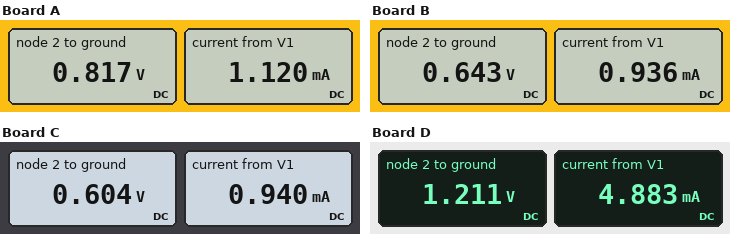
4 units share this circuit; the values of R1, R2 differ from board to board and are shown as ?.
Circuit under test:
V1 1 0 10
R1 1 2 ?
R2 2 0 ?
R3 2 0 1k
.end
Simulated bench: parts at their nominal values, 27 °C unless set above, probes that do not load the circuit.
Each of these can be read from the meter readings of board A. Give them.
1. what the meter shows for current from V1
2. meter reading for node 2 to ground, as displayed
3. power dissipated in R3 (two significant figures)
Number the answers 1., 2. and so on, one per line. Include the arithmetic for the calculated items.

1. 1.120 mA
2. 0.817 V
3. (817 mV)^2 / 1 kΩ = 670 µW
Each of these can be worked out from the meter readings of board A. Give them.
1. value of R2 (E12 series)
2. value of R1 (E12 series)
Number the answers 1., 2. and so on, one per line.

1. 2.7 kΩ
2. 8.2 kΩ
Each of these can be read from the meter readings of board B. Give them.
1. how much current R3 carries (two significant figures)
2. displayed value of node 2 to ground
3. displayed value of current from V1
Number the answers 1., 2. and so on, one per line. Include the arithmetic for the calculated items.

1. (643 mV) / 1 kΩ = 640 µA
2. 0.643 V
3. 0.936 mA
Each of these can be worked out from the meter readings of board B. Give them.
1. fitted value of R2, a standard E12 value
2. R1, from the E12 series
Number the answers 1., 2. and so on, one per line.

1. 2.2 kΩ
2. 10 kΩ
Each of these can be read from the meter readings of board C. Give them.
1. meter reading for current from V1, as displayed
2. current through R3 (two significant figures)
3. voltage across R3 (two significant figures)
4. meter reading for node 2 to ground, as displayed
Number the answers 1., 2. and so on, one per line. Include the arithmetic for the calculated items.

1. 0.940 mA
2. (604 mV) / 1 kΩ = 600 µA
3. 604 mV = 600 mV
4. 0.604 V
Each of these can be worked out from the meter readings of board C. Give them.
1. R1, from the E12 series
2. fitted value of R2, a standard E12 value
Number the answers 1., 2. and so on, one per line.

1. 10 kΩ
2. 1.8 kΩ
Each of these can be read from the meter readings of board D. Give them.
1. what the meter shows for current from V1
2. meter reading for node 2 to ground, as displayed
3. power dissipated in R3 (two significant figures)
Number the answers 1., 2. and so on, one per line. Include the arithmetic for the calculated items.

1. 4.883 mA
2. 1.211 V
3. (1.211 V)^2 / 1 kΩ = 1.5 mW
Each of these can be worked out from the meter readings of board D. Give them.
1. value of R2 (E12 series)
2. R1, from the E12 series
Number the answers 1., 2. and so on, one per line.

1. 330 Ω
2. 1.8 kΩ
